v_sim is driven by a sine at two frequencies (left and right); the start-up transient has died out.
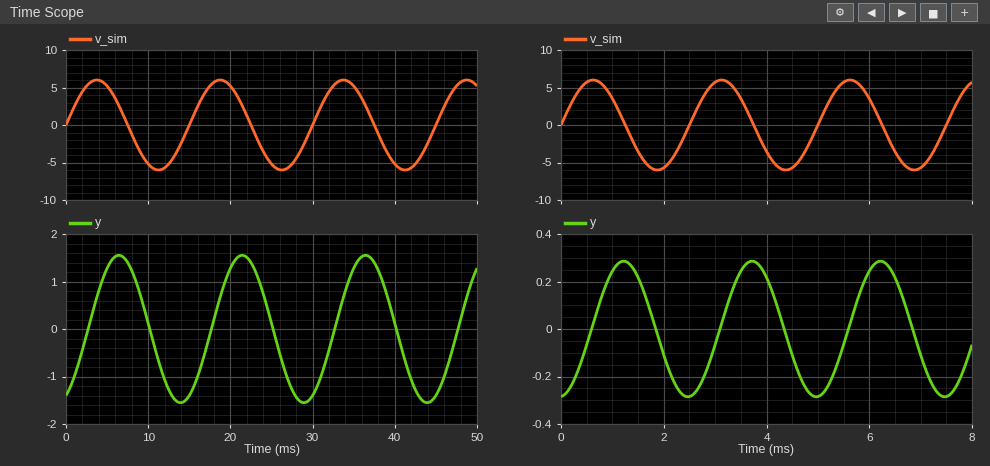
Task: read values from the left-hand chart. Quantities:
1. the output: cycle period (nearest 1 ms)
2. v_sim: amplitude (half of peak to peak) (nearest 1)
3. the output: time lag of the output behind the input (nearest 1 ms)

15 ms
6
3 ms
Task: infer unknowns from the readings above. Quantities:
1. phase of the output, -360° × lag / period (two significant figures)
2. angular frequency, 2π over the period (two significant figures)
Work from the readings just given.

-72°
0.42 rad/ms
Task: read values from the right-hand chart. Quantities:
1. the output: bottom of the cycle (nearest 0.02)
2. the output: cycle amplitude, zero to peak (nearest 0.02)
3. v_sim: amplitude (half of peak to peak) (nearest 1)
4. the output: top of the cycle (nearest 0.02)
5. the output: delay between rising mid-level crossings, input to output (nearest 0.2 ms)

-0.28
0.28
6
0.28
0.6 ms
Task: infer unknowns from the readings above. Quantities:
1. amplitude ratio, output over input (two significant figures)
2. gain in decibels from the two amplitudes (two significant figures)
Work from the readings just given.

0.047
-27 dB
